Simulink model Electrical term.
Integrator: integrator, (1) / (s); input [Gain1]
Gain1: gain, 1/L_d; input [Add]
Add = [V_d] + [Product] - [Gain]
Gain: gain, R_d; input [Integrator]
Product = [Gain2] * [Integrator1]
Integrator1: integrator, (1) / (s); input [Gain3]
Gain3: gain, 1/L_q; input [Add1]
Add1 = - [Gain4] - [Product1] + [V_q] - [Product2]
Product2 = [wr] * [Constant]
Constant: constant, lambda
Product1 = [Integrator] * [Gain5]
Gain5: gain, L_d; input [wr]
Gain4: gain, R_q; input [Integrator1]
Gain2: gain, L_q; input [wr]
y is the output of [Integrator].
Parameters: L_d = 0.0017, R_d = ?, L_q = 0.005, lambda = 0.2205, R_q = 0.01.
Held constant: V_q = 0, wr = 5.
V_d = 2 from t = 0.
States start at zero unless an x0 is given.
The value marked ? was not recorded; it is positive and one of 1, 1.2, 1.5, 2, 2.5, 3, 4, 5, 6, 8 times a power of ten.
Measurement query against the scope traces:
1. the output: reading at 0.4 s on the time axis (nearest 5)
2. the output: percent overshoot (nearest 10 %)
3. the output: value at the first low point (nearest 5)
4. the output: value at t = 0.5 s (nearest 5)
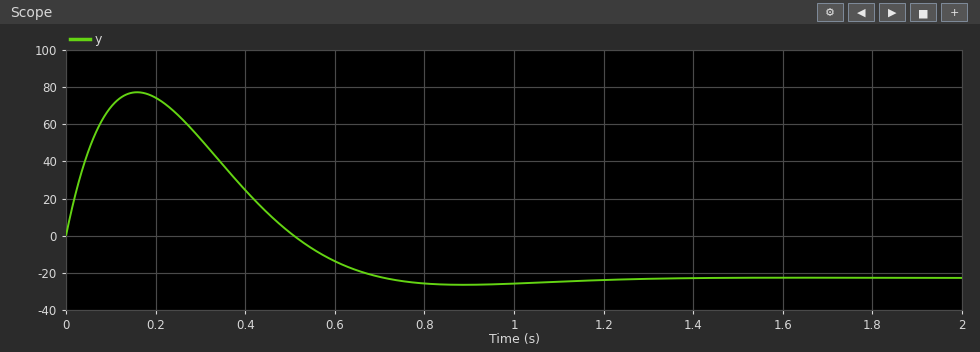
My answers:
25
20 %
-25
0
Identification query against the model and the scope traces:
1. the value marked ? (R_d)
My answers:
0.012
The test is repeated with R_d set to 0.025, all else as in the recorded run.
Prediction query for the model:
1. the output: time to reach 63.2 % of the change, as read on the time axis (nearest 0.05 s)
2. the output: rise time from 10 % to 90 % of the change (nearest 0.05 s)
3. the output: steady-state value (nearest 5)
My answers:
0.75 s
0.50 s
-15
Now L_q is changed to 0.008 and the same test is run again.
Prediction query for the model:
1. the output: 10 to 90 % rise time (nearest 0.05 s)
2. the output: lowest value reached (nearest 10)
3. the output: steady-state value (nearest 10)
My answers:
0.20 s
-60
-50
